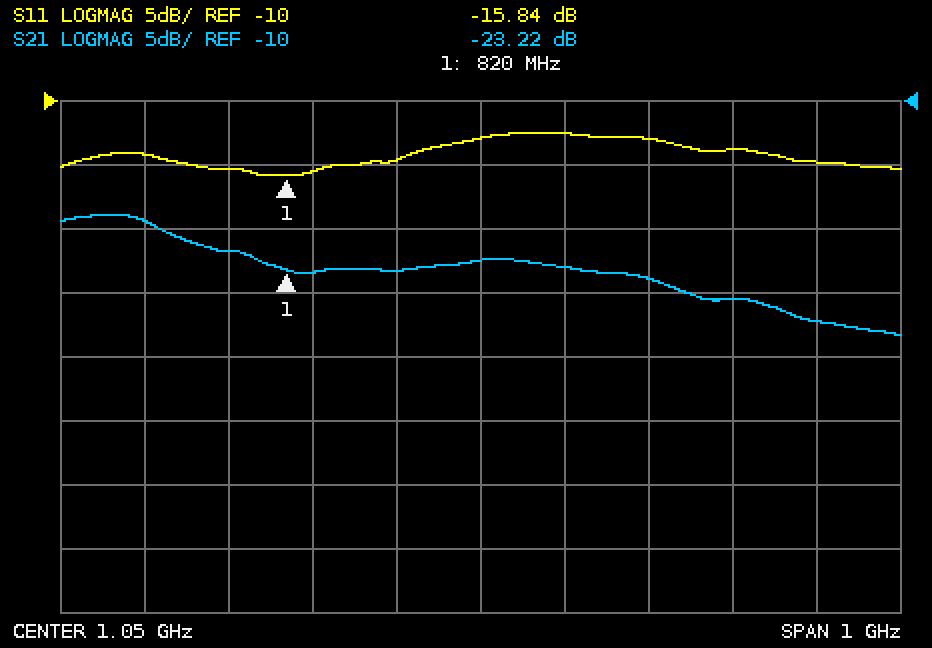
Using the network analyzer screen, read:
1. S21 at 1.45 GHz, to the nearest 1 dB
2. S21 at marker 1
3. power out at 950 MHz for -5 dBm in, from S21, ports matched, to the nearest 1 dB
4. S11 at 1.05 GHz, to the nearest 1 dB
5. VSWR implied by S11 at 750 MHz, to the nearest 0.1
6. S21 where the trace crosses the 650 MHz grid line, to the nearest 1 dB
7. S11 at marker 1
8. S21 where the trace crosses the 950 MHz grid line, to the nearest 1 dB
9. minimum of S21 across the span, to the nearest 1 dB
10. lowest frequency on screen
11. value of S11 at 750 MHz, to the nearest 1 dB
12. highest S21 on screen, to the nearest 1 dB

-27 dB
-23.22 dB
-28 dBm
-13 dB
1.4
-19 dB
-15.84 dB
-23 dB
-28 dB
550 MHz
-15 dB
-19 dB
